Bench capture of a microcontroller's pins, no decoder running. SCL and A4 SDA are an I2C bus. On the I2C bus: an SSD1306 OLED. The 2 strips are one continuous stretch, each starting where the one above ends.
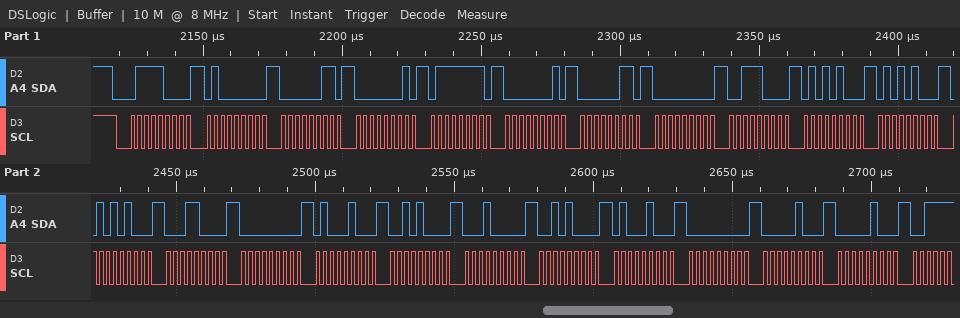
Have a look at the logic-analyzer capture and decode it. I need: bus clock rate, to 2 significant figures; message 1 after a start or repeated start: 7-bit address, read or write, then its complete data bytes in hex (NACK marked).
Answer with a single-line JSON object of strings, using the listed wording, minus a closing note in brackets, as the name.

{"bus clock rate, to 2 significant figures": "400 kHz", "message 1 after a start or repeated start: 7-bit address, read or write, then its complete data bytes in hex": "0x3C write: 40 03 01 7F 01 03 00 38 54 54 54 18 00 44 28 10 28 44 00 04 04"}
